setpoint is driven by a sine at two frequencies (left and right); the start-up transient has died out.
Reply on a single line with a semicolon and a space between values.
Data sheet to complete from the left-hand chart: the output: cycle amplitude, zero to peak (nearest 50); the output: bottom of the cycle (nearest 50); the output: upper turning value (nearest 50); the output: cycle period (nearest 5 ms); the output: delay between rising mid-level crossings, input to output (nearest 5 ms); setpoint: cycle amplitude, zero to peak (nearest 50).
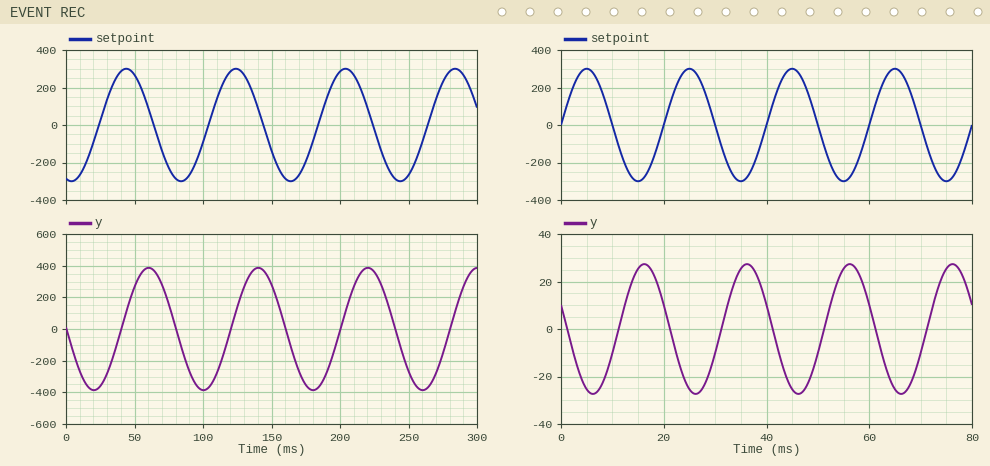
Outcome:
400; -400; 400; 80 ms; 15 ms; 300
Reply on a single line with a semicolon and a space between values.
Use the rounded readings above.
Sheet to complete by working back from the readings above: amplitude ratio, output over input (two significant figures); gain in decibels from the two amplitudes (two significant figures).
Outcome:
1.3; 2.5 dB
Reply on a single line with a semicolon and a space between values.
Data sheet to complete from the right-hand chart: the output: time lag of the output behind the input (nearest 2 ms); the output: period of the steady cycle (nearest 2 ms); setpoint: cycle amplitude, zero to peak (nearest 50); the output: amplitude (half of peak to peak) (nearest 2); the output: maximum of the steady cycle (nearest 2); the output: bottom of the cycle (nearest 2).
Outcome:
12 ms; 20 ms; 300; 28; 28; -28
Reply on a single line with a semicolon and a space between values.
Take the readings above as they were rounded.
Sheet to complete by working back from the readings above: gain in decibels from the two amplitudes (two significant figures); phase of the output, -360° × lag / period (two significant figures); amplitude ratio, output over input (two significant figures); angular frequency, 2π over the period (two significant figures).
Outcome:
-21 dB; -220°; 0.093; 0.31 rad/ms
